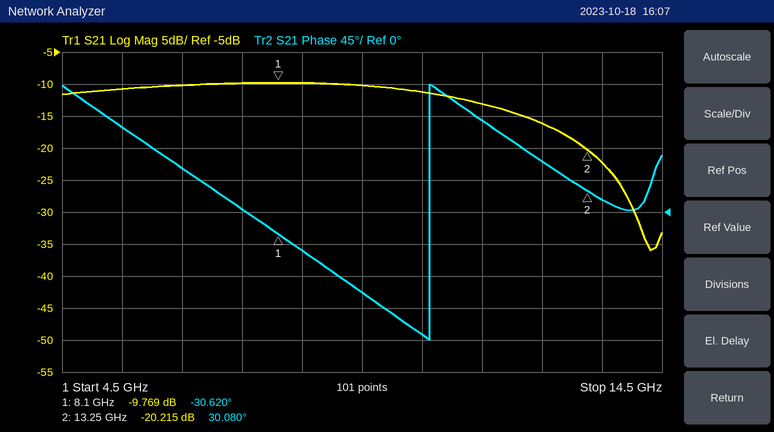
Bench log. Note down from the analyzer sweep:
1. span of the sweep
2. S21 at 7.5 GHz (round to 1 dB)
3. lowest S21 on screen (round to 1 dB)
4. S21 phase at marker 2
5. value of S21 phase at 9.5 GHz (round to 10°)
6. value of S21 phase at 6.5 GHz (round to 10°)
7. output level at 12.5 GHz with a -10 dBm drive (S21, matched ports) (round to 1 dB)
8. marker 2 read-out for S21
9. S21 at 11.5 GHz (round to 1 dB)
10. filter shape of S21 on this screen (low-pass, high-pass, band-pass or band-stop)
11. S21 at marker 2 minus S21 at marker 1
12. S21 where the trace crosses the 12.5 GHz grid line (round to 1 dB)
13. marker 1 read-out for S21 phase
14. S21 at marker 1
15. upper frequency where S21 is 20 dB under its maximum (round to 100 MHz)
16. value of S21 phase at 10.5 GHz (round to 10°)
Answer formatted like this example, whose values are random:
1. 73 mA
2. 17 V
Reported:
1. 10 GHz
2. -10 dB
3. -36 dB
4. 30.080°
5. -110°
6. 60°
7. -26 dBm
8. -20.215 dB
9. -13 dB
10. low-pass
11. -10.446 dB
12. -16 dB
13. -30.620°
14. -9.769 dB
15. 14.0 GHz
16. -170°
